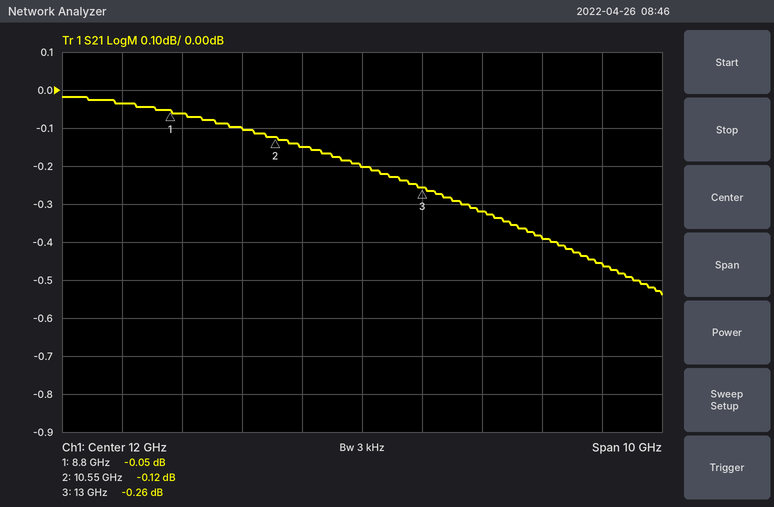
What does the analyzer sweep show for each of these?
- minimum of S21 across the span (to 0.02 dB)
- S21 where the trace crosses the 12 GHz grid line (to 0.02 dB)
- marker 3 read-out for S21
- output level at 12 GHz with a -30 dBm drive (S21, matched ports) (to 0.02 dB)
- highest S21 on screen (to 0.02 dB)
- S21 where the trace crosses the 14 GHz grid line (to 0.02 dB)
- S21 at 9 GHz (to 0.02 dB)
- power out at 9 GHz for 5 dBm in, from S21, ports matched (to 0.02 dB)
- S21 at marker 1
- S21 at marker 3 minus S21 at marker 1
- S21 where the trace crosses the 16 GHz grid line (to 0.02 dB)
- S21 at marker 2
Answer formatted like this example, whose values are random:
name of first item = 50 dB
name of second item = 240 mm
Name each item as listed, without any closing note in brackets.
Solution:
minimum of S21 across the span = -0.54 dB
S21 where the trace crosses the 12 GHz grid line = -0.20 dB
marker 3 read-out for S21 = -0.26 dB
output level at 12 GHz with a -30 dBm drive (S21, matched ports) = -30.20 dBm
highest S21 on screen = -0.02 dB
S21 where the trace crosses the 14 GHz grid line = -0.32 dB
S21 at 9 GHz = -0.06 dB
power out at 9 GHz for 5 dBm in, from S21, ports matched = 4.94 dBm
S21 at marker 1 = -0.05 dB
S21 at marker 3 minus S21 at marker 1 = -0.21 dB
S21 where the trace crosses the 16 GHz grid line = -0.46 dB
S21 at marker 2 = -0.12 dB
